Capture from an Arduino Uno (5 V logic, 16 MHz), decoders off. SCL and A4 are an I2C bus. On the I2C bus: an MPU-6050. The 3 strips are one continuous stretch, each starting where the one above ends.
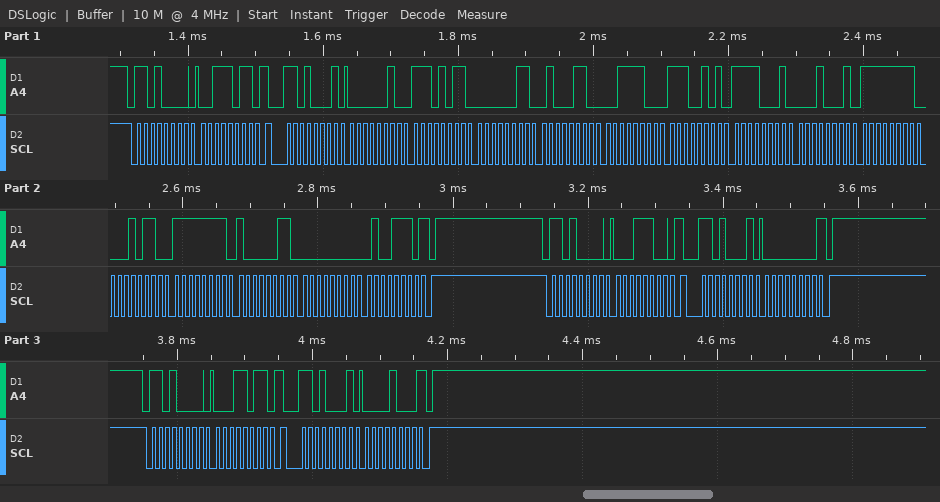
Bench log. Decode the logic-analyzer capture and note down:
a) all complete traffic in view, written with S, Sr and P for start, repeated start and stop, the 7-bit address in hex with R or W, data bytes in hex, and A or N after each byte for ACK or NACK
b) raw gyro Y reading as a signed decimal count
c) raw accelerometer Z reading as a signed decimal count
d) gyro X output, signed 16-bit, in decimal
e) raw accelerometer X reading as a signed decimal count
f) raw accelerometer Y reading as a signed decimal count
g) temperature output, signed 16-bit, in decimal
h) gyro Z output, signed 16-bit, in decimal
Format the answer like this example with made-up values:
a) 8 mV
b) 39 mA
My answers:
a) S 68W A 3B A Sr 68R A 02 A EB A 03 A 46 A 3C A E5 A F1 A 11 A FF A 16 A FF A 83 A 00 A 4E N P S 68W A 1C A Sr 68R A 00 N P S 68W A 1B A Sr 68R A 08 N P
b) -125
c) 15589
d) -234
e) 747
f) 838
g) -3823
h) 78
